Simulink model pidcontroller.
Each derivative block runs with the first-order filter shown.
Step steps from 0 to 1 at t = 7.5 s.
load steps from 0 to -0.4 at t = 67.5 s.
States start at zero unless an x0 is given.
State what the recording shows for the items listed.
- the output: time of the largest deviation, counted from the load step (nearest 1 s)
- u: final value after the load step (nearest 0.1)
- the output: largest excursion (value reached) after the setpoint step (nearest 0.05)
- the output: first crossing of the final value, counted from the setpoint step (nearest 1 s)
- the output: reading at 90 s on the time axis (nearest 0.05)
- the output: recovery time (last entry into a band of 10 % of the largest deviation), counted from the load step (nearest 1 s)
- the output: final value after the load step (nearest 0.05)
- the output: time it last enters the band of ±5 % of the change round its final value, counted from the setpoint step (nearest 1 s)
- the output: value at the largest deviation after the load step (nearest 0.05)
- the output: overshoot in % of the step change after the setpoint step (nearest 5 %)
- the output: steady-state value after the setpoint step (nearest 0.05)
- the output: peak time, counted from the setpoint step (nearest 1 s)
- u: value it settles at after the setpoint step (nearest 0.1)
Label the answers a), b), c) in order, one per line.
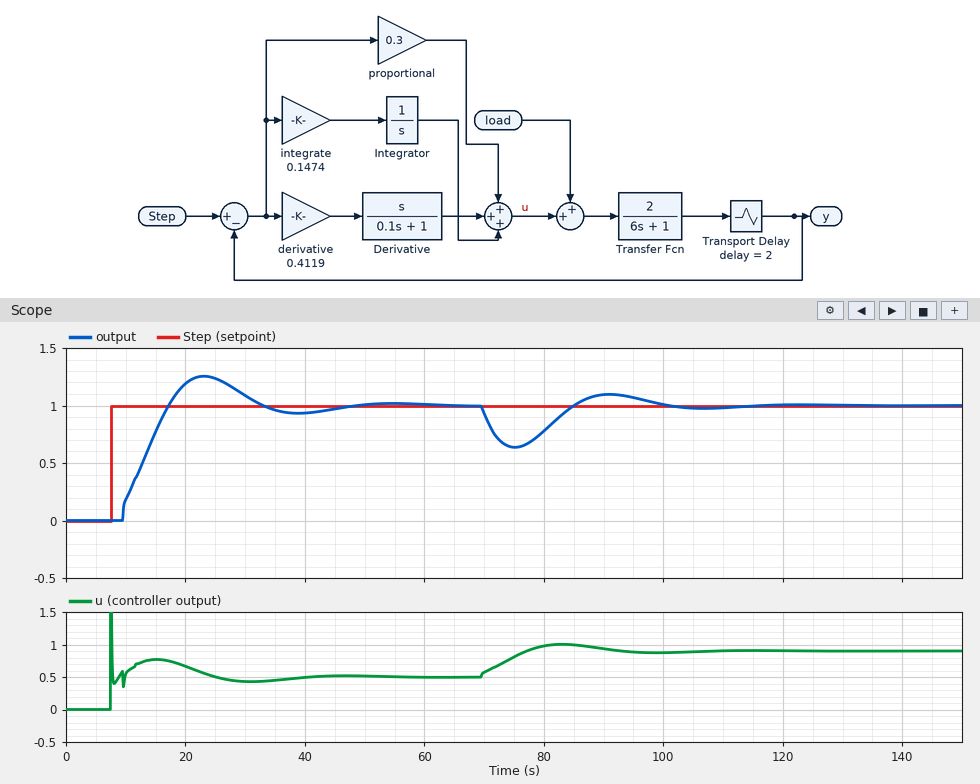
a) 8 s
b) 0.9
c) 1.25
d) 10 s
e) 1.10
f) 30 s
g) 1.00
h) 35 s
i) 0.65
j) 25 %
k) 1.00
l) 16 s
m) 0.5
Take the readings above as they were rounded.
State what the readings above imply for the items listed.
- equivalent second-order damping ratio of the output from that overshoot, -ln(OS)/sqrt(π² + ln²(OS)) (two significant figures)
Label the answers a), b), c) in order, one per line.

a) 0.40
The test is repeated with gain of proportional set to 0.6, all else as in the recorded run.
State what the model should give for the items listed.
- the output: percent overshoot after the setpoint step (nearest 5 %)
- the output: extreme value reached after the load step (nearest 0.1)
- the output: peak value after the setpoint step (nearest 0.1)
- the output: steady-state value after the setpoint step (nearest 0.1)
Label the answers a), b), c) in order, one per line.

a) 10 %
b) 0.7
c) 1.1
d) 1.0
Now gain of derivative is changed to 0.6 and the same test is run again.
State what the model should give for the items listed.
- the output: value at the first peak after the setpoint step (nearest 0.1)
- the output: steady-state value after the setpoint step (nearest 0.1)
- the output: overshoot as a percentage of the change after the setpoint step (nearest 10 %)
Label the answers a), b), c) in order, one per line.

a) 1.2
b) 1.0
c) 20 %
